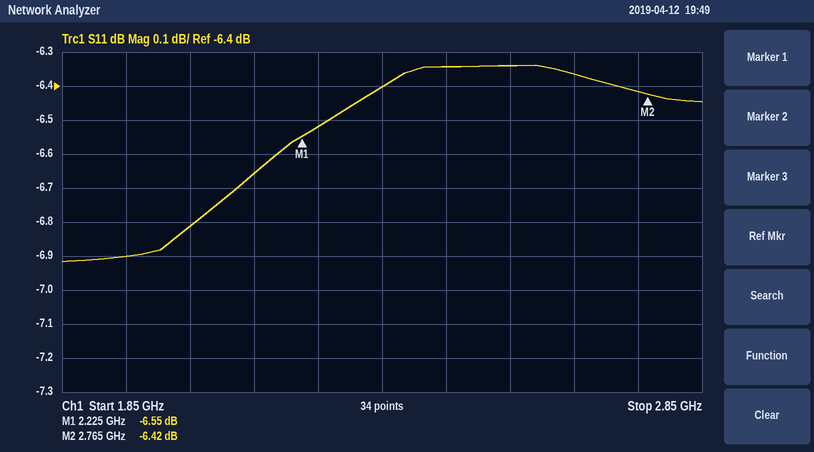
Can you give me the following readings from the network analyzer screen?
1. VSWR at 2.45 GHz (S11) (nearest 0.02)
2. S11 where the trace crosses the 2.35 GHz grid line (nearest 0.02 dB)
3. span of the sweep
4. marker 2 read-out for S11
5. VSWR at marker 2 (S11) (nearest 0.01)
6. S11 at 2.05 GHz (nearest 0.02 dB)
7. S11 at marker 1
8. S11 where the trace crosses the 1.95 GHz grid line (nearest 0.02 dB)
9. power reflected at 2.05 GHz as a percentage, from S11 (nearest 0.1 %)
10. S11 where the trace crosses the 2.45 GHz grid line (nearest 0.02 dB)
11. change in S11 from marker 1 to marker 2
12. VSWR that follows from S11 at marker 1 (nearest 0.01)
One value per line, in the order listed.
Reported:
2.86
-6.40 dB
1 GHz
-6.42 dB
2.83
-6.82 dB
-6.55 dB
-6.90 dB
20.8 %
-6.34 dB
0.13 dB
2.78
